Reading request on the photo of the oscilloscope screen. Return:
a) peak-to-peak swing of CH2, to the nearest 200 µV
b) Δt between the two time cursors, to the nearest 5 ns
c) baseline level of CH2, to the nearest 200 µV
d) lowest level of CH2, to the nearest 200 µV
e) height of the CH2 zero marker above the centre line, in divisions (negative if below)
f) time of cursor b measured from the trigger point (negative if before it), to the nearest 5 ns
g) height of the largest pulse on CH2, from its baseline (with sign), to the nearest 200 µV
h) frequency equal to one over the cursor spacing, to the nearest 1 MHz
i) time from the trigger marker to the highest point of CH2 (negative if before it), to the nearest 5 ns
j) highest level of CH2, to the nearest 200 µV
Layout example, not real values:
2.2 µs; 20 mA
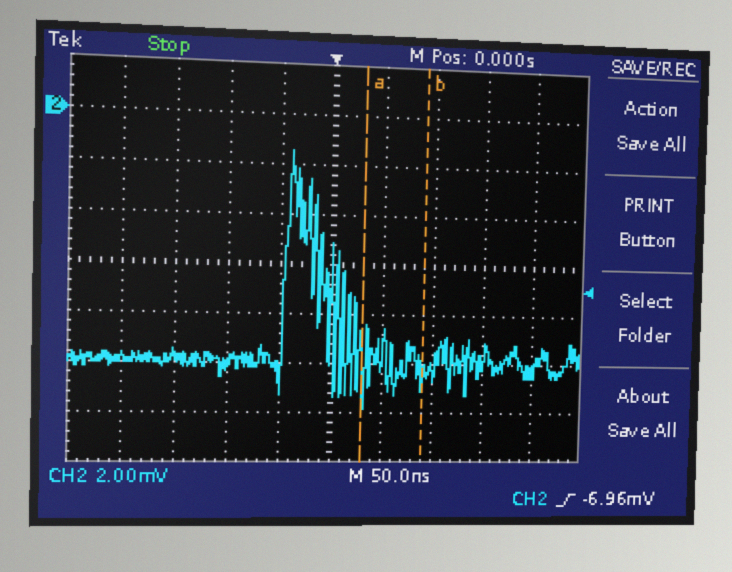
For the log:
10.4 mV; 60 ns; -9.8 mV; -11.8 mV; +3.0 div; +90 ns; +8.4 mV; 17 MHz; -40 ns; -1.4 mV
